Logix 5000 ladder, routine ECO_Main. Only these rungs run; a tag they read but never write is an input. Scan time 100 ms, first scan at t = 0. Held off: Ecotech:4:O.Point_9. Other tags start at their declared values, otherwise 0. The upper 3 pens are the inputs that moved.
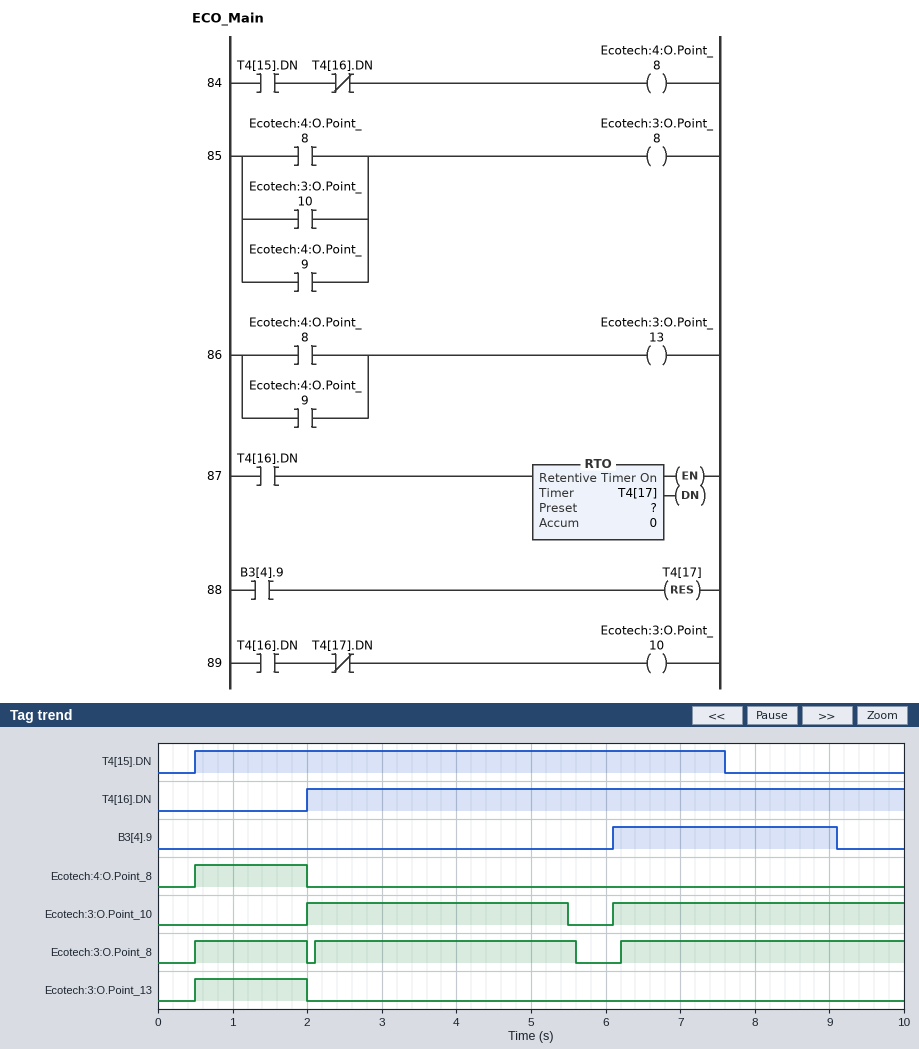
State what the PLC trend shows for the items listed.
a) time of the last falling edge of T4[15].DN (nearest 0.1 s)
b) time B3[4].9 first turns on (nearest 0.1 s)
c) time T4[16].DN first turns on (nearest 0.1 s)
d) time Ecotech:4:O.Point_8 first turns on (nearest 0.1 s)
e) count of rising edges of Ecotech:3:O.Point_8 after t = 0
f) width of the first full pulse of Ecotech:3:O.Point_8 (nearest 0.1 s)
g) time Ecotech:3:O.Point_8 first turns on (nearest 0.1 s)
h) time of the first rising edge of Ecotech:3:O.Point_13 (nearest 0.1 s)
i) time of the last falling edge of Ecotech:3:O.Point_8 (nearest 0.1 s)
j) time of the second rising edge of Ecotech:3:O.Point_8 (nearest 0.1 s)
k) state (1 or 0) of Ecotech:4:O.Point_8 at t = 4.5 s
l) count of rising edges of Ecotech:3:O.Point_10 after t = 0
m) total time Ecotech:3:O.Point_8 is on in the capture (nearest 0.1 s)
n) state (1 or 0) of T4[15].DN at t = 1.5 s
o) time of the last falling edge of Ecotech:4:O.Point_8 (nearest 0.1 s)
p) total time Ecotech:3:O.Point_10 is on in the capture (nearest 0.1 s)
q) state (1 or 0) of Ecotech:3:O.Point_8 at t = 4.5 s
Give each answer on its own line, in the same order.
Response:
7.6 s
6.1 s
2.0 s
0.5 s
3
1.5 s
0.5 s
0.5 s
5.6 s
2.1 s
0
2
8.8 s
1
2.0 s
7.4 s
1
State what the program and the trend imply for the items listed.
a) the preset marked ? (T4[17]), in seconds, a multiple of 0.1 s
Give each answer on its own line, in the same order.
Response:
3.5 s
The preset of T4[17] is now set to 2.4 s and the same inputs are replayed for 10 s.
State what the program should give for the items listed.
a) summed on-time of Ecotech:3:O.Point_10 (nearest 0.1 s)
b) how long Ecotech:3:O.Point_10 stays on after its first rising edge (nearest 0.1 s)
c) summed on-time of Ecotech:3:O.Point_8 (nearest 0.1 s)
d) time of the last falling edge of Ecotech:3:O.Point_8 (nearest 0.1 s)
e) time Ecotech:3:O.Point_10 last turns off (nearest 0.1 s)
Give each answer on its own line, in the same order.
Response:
6.3 s
2.4 s
7.7 s
4.5 s
4.4 s
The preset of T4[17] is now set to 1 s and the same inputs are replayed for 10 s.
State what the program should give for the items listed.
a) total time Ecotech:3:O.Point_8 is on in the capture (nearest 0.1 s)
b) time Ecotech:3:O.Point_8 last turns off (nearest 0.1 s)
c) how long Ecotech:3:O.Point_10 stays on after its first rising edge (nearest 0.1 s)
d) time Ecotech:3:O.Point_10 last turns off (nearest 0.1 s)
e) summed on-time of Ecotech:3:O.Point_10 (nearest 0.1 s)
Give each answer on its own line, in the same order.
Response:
6.3 s
3.1 s
1.0 s
3.0 s
4.9 s
